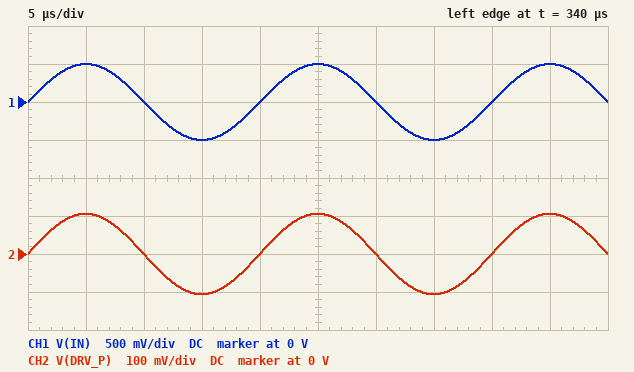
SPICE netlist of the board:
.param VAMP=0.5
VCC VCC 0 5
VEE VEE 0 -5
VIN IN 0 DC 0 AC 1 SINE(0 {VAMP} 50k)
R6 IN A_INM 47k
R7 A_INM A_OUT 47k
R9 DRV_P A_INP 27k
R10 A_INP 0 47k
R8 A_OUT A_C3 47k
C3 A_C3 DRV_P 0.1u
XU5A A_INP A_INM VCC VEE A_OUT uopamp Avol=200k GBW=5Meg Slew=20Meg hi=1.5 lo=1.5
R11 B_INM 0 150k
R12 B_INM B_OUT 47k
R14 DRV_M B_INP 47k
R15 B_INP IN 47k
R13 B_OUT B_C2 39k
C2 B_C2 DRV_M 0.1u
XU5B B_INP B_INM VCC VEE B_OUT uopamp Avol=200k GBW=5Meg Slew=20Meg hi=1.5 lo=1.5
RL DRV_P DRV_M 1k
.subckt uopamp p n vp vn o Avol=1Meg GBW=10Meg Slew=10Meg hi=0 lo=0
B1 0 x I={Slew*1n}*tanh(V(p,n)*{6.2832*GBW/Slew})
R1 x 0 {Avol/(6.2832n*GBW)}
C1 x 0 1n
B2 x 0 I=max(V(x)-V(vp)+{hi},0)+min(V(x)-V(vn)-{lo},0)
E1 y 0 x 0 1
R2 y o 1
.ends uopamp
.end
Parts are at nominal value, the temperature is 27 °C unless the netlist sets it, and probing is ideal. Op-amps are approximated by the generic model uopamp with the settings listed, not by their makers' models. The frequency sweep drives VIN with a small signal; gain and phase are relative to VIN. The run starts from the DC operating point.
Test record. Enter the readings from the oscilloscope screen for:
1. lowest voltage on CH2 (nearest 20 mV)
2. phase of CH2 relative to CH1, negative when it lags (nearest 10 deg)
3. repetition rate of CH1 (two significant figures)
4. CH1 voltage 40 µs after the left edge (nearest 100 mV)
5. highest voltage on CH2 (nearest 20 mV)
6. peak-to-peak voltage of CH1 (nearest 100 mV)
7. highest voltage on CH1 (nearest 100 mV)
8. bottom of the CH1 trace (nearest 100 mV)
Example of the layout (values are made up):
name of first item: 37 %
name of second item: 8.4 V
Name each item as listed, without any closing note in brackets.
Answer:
lowest voltage on CH2: -100 mV
phase of CH2 relative to CH1, negative when it lags: 0 deg
repetition rate of CH1: 50 kHz
CH1 voltage 40 µs after the left edge: 0 V
highest voltage on CH2: 100 mV
peak-to-peak voltage of CH1: 1.0 V
highest voltage on CH1: 500 mV
bottom of the CH1 trace: -500 mV
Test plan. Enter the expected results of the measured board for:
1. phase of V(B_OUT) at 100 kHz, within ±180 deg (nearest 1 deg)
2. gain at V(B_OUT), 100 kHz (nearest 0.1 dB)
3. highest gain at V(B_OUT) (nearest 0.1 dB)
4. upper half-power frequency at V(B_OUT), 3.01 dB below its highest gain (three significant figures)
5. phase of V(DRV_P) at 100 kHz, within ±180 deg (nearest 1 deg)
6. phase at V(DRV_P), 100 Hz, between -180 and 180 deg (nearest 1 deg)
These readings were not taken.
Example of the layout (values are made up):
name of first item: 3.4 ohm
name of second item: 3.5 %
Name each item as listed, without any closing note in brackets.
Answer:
phase of V(B_OUT) at 100 kHz, within ±180 deg: -1 deg
gain at V(B_OUT), 100 kHz: -1.8 dB
highest gain at V(B_OUT): -0.5 dB
upper half-power frequency at V(B_OUT), 3.01 dB below its highest gain: 2.64 MHz
phase of V(DRV_P) at 100 kHz, within ±180 deg: 1 deg
phase at V(DRV_P), 100 Hz, between -180 and 180 deg: -10 deg
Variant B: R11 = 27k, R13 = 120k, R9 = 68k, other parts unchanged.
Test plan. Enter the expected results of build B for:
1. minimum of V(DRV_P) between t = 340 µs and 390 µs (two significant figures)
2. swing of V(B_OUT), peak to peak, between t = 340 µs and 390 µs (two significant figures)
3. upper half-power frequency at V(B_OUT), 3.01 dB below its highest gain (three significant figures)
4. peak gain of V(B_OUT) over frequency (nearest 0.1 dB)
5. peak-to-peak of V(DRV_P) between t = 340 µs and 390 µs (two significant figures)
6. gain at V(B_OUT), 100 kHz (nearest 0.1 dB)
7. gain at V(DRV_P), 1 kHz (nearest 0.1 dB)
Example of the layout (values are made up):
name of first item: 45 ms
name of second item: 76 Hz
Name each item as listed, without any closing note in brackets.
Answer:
minimum of V(DRV_P) between t = 340 µs and 390 µs: -15 mV
swing of V(B_OUT), peak to peak, between t = 340 µs and 390 µs: 1.4 V
upper half-power frequency at V(B_OUT), 3.01 dB below its highest gain: 76.0 Hz
peak gain of V(B_OUT) over frequency: 7.6 dB
peak-to-peak of V(DRV_P) between t = 340 µs and 390 µs: 31 mV
gain at V(B_OUT), 100 kHz: 3.2 dB
gain at V(DRV_P), 1 kHz: -27.4 dB
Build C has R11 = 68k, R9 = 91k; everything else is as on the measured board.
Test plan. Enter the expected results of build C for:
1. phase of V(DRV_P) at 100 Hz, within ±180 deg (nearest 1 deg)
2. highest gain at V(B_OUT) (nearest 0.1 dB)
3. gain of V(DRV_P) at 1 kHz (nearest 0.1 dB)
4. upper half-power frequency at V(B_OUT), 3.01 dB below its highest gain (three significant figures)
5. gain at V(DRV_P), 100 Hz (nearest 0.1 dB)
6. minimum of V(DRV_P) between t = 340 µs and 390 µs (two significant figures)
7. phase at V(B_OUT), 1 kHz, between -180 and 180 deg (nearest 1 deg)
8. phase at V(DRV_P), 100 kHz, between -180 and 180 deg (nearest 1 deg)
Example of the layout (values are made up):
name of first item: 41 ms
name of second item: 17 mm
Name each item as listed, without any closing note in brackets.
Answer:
phase of V(DRV_P) at 100 Hz, within ±180 deg: -1 deg
highest gain at V(B_OUT): 2.6 dB
gain of V(DRV_P) at 1 kHz: -8.6 dB
upper half-power frequency at V(B_OUT), 3.01 dB below its highest gain: 1.66 MHz
gain at V(DRV_P), 100 Hz: -8.9 dB
minimum of V(DRV_P) between t = 340 µs and 390 µs: -190 mV
phase at V(B_OUT), 1 kHz, between -180 and 180 deg: 0 deg
phase at V(DRV_P), 100 kHz, between -180 and 180 deg: -2 deg
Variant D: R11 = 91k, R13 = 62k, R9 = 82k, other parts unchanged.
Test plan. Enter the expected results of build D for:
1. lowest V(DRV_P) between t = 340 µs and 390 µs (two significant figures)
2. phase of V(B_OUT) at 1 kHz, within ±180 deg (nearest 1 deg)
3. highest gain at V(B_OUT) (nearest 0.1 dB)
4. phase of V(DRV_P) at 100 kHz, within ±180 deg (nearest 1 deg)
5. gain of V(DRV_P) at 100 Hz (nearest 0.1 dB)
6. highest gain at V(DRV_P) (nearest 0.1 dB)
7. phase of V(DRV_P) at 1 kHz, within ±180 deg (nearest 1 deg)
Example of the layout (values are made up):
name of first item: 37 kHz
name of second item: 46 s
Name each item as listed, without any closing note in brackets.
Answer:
lowest V(DRV_P) between t = 340 µs and 390 µs: -23 mV
phase of V(B_OUT) at 1 kHz, within ±180 deg: -1 deg
highest gain at V(B_OUT): 1.6 dB
phase of V(DRV_P) at 100 kHz, within ±180 deg: 18 deg
gain of V(DRV_P) at 100 Hz: -15.6 dB
highest gain at V(DRV_P): -4.8 dB
phase of V(DRV_P) at 1 kHz, within ±180 deg: -18 deg
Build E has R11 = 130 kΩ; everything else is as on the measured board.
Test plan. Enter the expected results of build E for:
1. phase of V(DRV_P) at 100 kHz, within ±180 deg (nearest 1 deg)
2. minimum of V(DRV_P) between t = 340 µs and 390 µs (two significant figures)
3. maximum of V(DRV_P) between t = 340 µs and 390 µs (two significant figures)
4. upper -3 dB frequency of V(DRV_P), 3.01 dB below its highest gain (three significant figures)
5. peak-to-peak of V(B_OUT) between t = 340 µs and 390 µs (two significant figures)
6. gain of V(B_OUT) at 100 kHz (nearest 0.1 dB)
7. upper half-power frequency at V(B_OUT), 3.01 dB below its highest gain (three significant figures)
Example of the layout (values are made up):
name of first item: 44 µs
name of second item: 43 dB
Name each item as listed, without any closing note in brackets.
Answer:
phase of V(DRV_P) at 100 kHz, within ±180 deg: 0 deg
minimum of V(DRV_P) between t = 340 µs and 390 µs: -120 mV
maximum of V(DRV_P) between t = 340 µs and 390 µs: 120 mV
upper -3 dB frequency of V(DRV_P), 3.01 dB below its highest gain: 30.6 Hz
peak-to-peak of V(B_OUT) between t = 340 µs and 390 µs: 860 mV
gain of V(B_OUT) at 100 kHz: -1.3 dB
upper half-power frequency at V(B_OUT), 3.01 dB below its highest gain: 2.55 MHz
